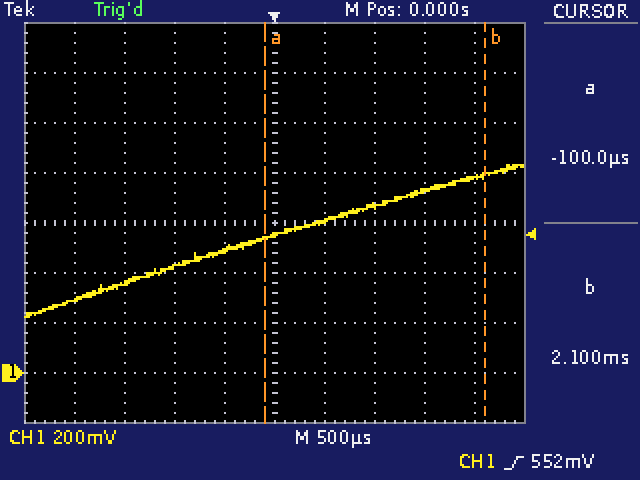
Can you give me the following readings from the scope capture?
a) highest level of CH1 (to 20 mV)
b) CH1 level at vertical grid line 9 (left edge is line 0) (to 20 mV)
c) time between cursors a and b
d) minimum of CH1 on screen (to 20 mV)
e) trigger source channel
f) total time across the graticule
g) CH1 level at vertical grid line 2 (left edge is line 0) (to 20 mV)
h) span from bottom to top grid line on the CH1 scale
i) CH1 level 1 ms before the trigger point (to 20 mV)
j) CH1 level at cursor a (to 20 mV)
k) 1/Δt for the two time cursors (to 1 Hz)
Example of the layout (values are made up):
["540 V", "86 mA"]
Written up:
["840 mV", "780 mV", "2.20 ms", "220 mV", "CH1", "5 ms", "360 mV", "1.6 V", "420 mV", "540 mV", "455 Hz"]
